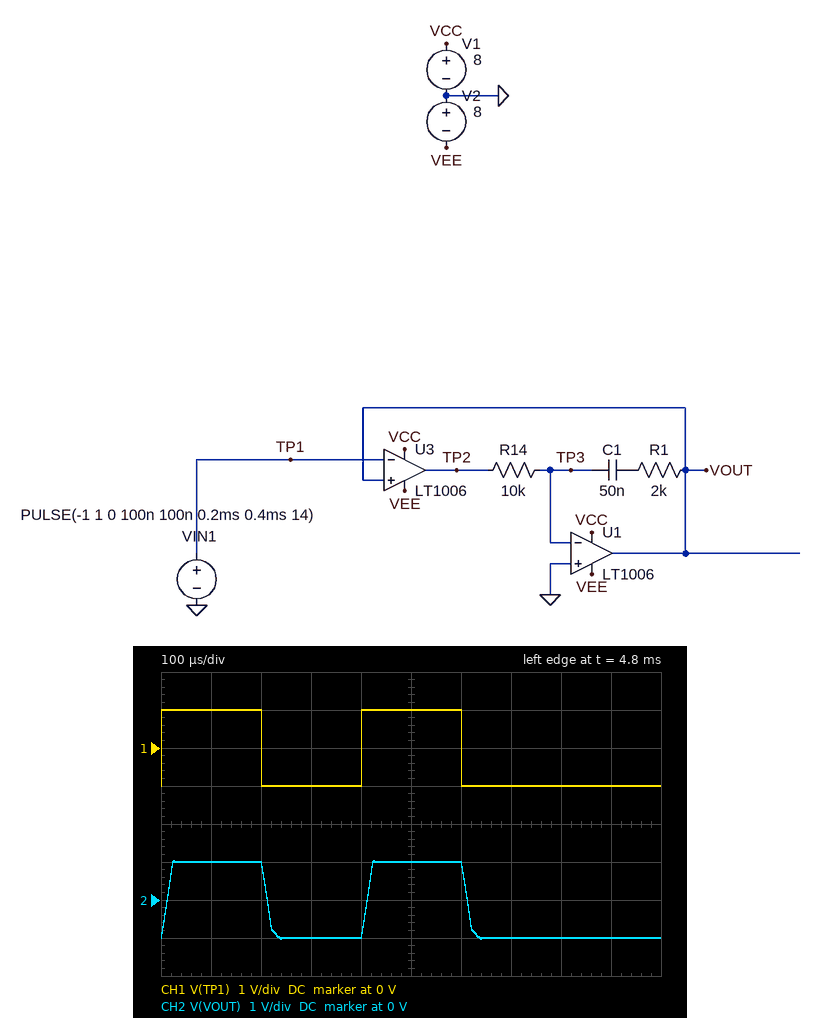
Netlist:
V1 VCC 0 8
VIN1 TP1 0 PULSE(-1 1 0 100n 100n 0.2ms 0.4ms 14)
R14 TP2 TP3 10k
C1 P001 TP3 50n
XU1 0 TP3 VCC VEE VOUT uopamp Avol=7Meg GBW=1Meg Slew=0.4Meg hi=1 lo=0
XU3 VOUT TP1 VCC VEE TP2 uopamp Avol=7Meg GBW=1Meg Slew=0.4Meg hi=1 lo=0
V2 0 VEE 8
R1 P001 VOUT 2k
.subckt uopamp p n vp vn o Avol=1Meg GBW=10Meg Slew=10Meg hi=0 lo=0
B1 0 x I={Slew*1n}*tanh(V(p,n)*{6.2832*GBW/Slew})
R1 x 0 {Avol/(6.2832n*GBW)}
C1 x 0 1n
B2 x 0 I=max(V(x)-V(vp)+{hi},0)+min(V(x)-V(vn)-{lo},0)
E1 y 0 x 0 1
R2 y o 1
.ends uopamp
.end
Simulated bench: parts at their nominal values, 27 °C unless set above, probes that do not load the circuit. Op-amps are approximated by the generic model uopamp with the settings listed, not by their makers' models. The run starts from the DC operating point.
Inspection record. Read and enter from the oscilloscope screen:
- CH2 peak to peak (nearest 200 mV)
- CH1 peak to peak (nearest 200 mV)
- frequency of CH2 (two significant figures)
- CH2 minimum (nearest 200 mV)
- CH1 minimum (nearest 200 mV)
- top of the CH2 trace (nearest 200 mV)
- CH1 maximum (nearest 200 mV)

2.0 V
2.0 V
2.5 kHz
-1.0 V
-1.0 V
1.0 V
1.0 V
